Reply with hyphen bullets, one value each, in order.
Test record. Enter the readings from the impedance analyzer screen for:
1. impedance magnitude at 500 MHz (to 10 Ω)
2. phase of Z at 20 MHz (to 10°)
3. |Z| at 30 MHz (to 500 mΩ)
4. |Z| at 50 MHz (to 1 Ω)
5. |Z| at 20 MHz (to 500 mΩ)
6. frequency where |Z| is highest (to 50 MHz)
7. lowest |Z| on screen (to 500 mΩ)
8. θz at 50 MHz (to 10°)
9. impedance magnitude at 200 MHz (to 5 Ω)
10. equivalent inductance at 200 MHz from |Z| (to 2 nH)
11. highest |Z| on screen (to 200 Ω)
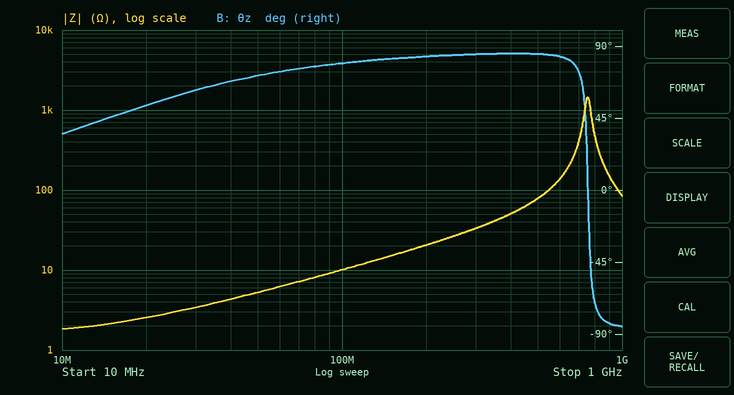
- 80 Ω
- 50°
- 3.5 Ω
- 5 Ω
- 2.5 Ω
- 750 MHz
- 2.0 Ω
- 70°
- 20 Ω
- 16 nH
- 1.4 kΩ
